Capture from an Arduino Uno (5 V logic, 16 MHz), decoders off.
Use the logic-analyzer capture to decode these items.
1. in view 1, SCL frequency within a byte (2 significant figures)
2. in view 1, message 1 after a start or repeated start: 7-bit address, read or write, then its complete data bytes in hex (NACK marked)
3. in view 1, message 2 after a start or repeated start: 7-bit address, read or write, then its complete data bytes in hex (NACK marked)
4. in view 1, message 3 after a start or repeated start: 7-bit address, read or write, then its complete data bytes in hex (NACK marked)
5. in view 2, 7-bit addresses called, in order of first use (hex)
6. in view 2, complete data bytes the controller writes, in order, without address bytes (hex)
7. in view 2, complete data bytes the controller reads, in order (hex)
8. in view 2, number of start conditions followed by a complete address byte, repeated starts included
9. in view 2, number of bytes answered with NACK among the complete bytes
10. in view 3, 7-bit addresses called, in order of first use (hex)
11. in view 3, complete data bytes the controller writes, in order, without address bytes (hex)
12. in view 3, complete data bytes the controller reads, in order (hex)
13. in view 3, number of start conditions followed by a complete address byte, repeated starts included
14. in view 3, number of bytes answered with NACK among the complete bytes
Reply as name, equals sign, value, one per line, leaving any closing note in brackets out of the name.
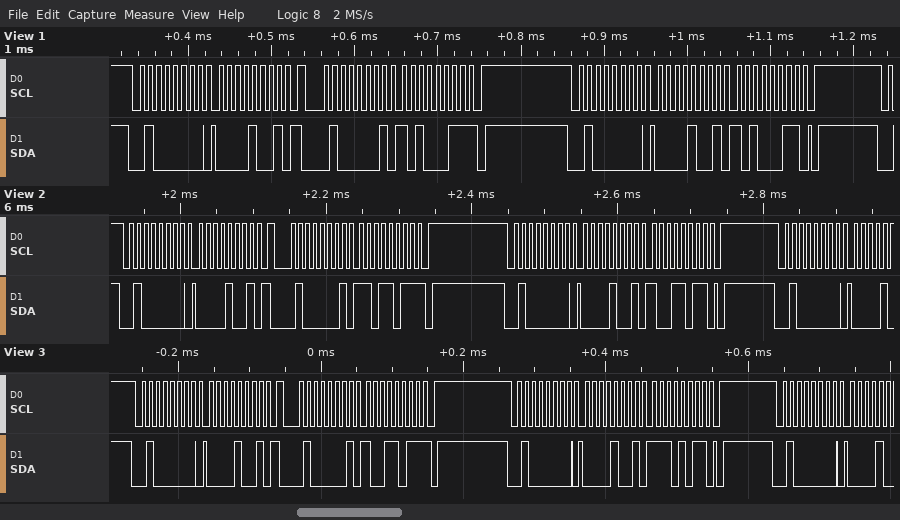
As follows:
in view 1, SCL frequency within a byte = 100 kHz
in view 1, message 1 after a start or repeated start: 7-bit address, read or write, then its complete data bytes in hex = 0x20 write: 09
in view 1, message 2 after a start or repeated start: 7-bit address, read or write, then its complete data bytes in hex = 0x20 read: A3 NACK
in view 1, message 3 after a start or repeated start: 7-bit address, read or write, then its complete data bytes in hex = 0x20 write: 09 A3
in view 2, 7-bit addresses called, in order of first use = 0x20
in view 2, complete data bytes the controller writes, in order, without address bytes = 09 09 9B
in view 2, complete data bytes the controller reads, in order = DB
in view 2, number of start conditions followed by a complete address byte, repeated starts included = 4
in view 2, number of bytes answered with NACK among the complete bytes = 1
in view 3, 7-bit addresses called, in order of first use = 0x20
in view 3, complete data bytes the controller writes, in order, without address bytes = 09 09 EB
in view 3, complete data bytes the controller reads, in order = 9B
in view 3, number of start conditions followed by a complete address byte, repeated starts included = 4
in view 3, number of bytes answered with NACK among the complete bytes = 1
